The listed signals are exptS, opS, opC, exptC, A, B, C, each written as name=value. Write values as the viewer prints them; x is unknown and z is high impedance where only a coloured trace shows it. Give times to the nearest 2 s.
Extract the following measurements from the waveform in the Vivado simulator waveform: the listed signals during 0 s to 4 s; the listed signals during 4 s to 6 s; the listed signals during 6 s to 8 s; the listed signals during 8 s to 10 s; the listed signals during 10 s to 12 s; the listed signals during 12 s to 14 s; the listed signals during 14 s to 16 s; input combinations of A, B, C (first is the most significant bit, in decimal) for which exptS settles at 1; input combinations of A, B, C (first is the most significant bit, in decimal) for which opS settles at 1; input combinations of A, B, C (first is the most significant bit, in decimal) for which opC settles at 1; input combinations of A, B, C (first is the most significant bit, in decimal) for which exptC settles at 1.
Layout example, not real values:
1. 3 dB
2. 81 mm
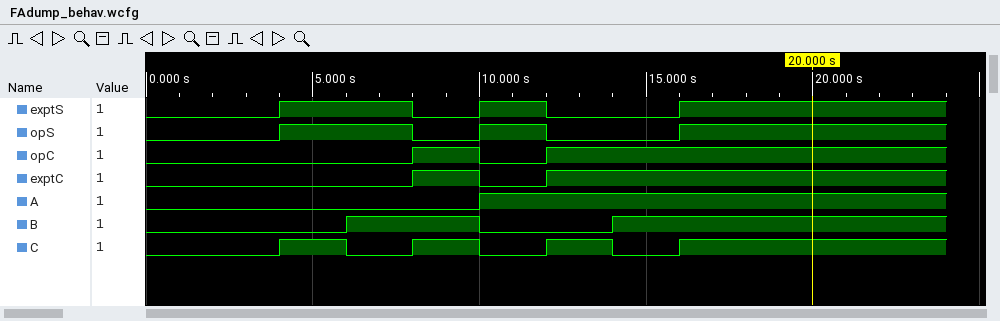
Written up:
1. exptS=0, opS=0, opC=0, exptC=0, A=0, B=0, C=0
2. exptS=1, opS=1, opC=0, exptC=0, A=0, B=0, C=1
3. exptS=1, opS=1, opC=0, exptC=0, A=0, B=1, C=0
4. exptS=0, opS=0, opC=1, exptC=1, A=0, B=1, C=1
5. exptS=1, opS=1, opC=0, exptC=0, A=1, B=0, C=0
6. exptS=0, opS=0, opC=1, exptC=1, A=1, B=0, C=1
7. exptS=0, opS=0, opC=1, exptC=1, A=1, B=1, C=0
8. 1, 2, 4, 7
9. 1, 2, 4, 7
10. 3, 5, 6, 7
11. 3, 5, 6, 7
